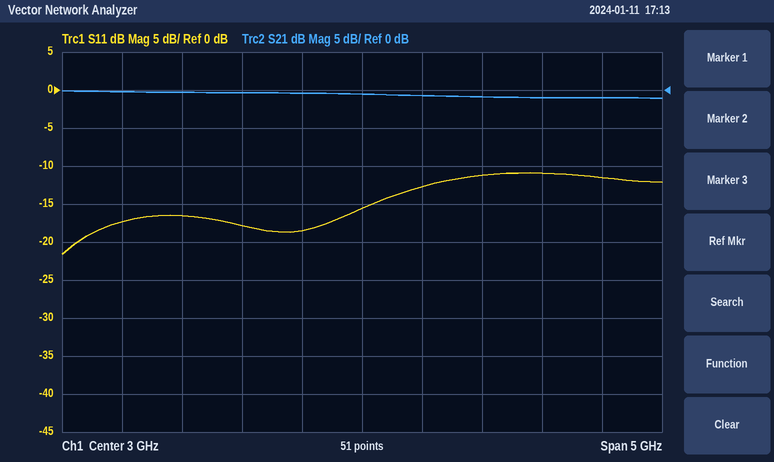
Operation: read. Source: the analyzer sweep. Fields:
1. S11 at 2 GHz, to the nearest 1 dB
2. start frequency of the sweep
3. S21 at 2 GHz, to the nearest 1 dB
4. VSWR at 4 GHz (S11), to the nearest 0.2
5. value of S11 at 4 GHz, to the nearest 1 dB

-18 dB
500 MHz
0 dB
1.8
-11 dB
